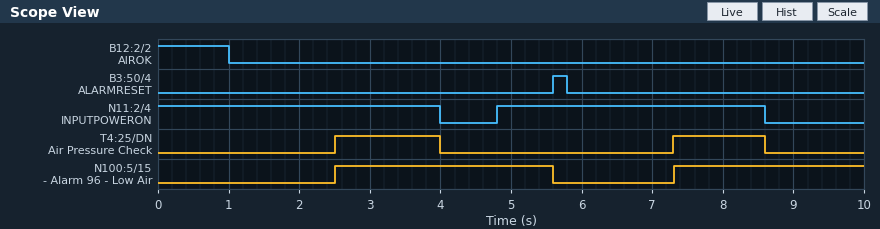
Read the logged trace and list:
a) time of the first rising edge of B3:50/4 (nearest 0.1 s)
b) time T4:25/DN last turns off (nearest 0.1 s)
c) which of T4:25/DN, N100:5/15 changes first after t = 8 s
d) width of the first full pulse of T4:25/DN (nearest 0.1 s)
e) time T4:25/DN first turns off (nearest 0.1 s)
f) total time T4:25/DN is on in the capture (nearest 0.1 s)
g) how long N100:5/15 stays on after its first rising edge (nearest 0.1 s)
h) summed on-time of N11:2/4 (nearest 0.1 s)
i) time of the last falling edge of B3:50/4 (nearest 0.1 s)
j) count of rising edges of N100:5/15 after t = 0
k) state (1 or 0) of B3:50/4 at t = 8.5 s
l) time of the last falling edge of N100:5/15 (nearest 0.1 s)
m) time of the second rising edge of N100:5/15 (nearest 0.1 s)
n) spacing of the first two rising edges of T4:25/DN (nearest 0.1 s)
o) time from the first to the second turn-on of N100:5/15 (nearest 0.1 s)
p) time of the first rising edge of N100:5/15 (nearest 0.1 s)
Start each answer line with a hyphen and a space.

- 5.6 s
- 8.6 s
- T4:25/DN
- 1.5 s
- 4.0 s
- 2.8 s
- 3.1 s
- 7.8 s
- 5.8 s
- 2
- 0
- 5.6 s
- 7.3 s
- 4.8 s
- 4.8 s
- 2.5 s
